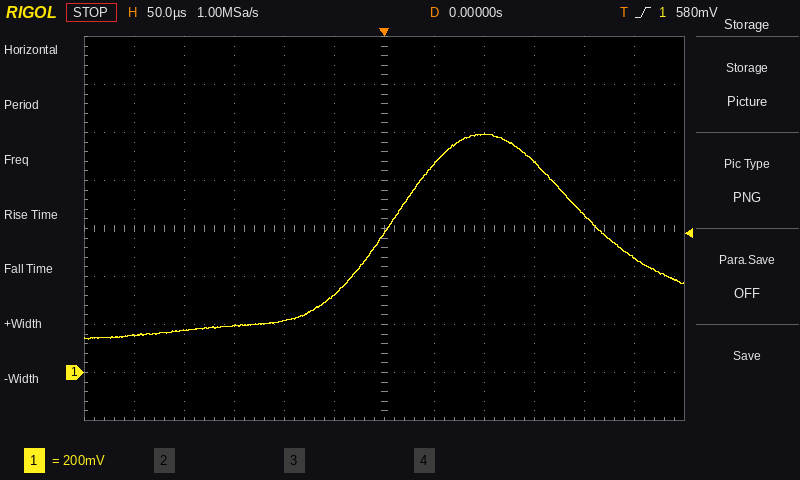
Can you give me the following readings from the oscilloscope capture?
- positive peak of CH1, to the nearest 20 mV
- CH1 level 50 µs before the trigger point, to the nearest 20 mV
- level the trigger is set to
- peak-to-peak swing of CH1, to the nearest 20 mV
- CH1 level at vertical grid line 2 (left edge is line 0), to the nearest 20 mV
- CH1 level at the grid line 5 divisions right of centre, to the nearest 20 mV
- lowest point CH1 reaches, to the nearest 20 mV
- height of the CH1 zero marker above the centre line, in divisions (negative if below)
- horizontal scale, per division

1.00 V
320 mV
580 mV
860 mV
180 mV
480 mV
140 mV
-3.0 div
50 µs
